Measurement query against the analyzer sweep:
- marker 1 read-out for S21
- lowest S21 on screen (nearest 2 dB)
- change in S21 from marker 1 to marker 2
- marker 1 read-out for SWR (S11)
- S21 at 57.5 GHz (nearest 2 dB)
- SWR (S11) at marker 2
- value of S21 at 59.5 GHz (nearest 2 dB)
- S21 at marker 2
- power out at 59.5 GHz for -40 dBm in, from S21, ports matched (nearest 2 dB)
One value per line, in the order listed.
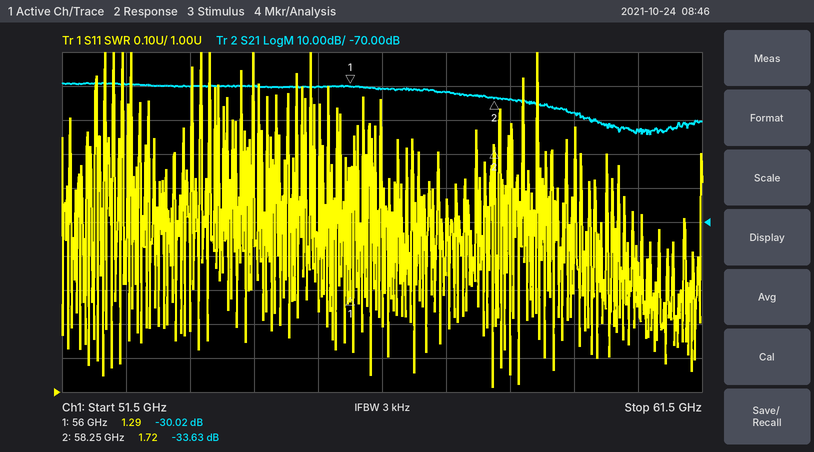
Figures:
-30.02 dB
-44 dB
-3.61 dB
1.29
-32 dB
1.72
-38 dB
-33.63 dB
-78 dBm
